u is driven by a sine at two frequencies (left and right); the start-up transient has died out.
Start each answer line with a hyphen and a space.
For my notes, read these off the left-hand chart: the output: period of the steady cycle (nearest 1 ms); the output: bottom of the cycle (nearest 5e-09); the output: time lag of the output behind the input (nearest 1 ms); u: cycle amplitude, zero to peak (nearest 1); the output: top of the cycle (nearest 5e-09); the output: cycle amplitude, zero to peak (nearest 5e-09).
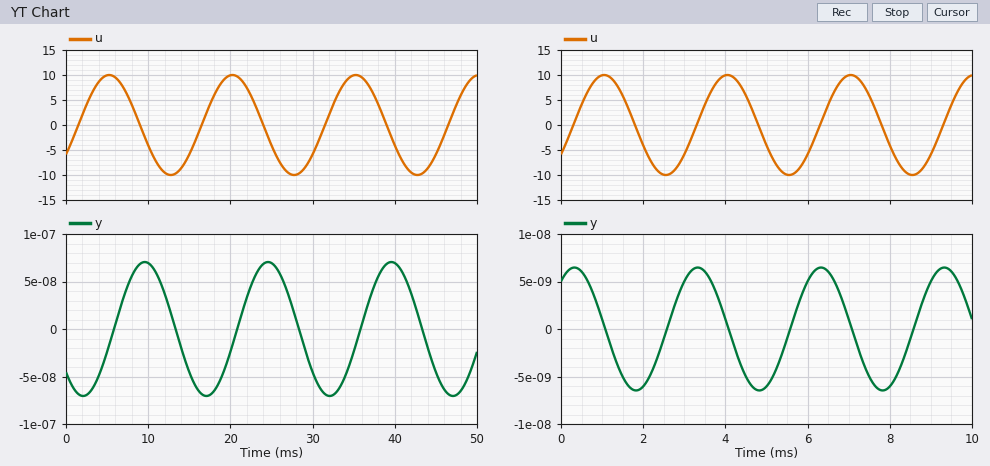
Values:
- 15 ms
- -0.000000070
- 4 ms
- 10
- 0.000000070
- 0.000000070
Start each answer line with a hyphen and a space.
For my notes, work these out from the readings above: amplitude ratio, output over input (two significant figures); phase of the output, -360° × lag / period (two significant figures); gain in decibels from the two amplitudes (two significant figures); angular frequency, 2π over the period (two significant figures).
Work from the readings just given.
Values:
- 0.0000000070
- -96°
- -160 dB
- 0.42 rad/ms
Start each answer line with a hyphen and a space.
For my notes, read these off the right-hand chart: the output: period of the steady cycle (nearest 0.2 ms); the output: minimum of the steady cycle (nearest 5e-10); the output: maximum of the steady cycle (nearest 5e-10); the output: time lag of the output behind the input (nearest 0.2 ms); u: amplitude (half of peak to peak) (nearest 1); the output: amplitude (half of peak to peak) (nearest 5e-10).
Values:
- 3.0 ms
- -0.0000000065
- 0.0000000065
- 2.2 ms
- 10
- 0.0000000065
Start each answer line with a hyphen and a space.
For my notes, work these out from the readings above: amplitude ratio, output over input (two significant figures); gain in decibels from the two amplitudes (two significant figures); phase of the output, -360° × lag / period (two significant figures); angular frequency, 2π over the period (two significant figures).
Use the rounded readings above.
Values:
- 0.00000000065
- -180 dB
- -260°
- 2.1 rad/ms
